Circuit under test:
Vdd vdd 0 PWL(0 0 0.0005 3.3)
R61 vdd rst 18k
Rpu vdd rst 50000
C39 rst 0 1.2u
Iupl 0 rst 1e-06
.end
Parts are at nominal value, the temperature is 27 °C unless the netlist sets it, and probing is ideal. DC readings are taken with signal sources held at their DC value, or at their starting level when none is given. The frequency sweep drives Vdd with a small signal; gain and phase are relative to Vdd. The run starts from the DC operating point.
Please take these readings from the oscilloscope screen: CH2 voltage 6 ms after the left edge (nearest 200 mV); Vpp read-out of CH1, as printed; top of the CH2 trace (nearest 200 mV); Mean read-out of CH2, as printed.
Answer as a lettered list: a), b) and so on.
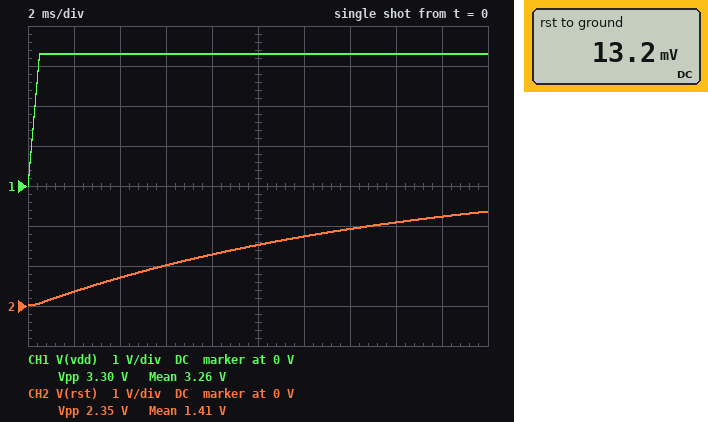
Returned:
a) 1.0 V
b) 3.30 V
c) 2.4 V
d) 1.41 V
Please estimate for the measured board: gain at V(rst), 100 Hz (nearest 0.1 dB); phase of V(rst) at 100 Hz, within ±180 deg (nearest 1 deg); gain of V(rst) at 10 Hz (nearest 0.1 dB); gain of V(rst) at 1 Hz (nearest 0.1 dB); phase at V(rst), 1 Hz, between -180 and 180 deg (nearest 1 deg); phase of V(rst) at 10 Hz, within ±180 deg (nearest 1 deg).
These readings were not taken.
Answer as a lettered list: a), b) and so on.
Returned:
a) -20.0 dB
b) -84 deg
c) -3.0 dB
d) 0 dB
e) -6 deg
f) -45 deg
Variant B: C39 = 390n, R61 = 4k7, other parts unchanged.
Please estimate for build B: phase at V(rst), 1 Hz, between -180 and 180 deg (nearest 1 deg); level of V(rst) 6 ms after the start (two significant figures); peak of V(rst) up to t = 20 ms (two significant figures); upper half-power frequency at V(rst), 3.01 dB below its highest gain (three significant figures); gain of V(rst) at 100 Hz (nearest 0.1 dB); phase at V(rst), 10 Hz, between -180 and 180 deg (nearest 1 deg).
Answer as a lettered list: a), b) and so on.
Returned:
a) -1 deg
b) 3.2 V
c) 3.3 V
d) 95.0 Hz
e) -3.2 dB
f) -6 deg
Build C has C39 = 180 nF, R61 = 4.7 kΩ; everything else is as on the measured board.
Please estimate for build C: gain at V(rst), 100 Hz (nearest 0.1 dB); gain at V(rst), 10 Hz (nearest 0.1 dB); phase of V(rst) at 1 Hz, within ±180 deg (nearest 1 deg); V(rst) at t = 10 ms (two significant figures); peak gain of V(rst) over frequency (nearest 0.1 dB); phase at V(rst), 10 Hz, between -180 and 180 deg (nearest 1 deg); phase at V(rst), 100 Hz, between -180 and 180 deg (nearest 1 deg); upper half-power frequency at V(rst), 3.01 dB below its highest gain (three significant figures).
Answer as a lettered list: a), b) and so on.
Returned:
a) -0.9 dB
b) 0 dB
c) 0 deg
d) 3.3 V
e) 0 dB
f) -3 deg
g) -26 deg
h) 206 Hz
